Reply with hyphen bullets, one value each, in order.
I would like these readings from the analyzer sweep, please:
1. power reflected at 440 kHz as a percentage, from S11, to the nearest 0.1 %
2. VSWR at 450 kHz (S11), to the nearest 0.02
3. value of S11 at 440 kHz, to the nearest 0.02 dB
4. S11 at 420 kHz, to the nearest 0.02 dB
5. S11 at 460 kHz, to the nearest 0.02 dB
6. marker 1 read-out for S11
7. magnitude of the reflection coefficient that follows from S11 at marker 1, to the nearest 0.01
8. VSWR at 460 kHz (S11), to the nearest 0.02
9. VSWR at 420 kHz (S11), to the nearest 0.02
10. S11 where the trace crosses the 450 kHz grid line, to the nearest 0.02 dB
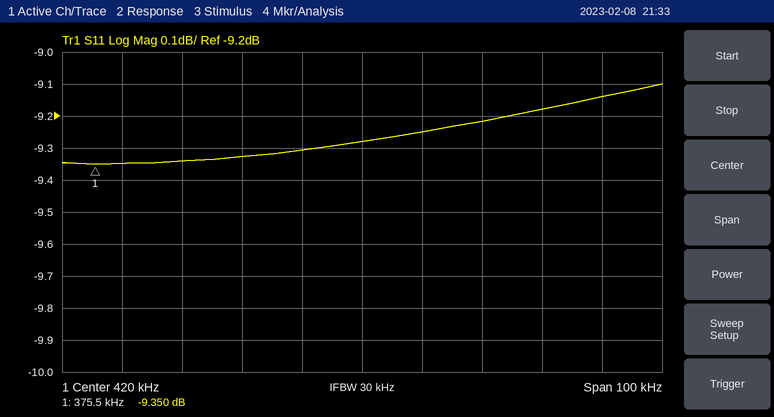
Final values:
- 12.0 %
- 2.06
- -9.22 dB
- -9.28 dB
- -9.14 dB
- -9.350 dB
- 0.34
- 2.08
- 2.04
- -9.18 dB
